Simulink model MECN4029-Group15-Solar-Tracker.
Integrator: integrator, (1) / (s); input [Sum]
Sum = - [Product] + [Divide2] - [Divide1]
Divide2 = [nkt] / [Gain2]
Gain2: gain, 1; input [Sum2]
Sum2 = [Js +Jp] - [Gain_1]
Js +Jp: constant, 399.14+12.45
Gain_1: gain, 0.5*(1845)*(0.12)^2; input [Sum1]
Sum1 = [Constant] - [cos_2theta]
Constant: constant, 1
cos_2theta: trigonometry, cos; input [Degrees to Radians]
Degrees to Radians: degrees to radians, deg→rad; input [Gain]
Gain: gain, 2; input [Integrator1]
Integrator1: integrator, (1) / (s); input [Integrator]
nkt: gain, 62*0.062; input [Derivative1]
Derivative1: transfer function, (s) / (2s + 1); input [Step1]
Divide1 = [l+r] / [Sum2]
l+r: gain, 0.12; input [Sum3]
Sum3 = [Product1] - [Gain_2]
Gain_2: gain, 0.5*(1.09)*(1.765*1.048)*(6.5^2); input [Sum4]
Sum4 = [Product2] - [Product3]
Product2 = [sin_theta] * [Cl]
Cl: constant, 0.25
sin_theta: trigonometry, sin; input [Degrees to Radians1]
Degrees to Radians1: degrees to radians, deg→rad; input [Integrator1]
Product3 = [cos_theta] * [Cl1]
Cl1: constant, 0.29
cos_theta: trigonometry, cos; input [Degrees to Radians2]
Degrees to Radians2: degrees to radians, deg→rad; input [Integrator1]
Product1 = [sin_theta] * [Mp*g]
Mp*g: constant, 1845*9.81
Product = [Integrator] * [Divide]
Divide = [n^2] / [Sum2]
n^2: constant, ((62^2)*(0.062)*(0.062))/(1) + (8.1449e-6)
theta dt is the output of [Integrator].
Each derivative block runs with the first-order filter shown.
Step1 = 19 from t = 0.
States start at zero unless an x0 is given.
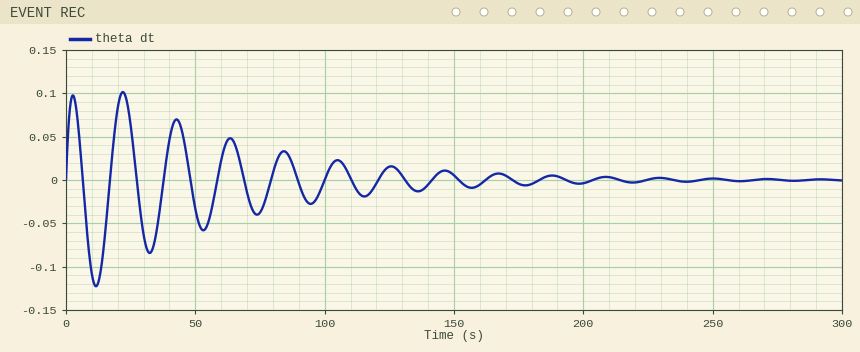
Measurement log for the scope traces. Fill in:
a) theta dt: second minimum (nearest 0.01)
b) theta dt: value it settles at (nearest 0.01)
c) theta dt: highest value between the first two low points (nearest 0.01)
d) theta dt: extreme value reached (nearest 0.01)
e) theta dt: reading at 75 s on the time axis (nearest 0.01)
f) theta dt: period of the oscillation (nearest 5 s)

-0.08
0.00
0.10
-0.12
-0.04
20 s
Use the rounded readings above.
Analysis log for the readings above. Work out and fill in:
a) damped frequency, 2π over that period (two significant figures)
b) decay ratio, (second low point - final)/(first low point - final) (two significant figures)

0.31 rad/s
0.67
